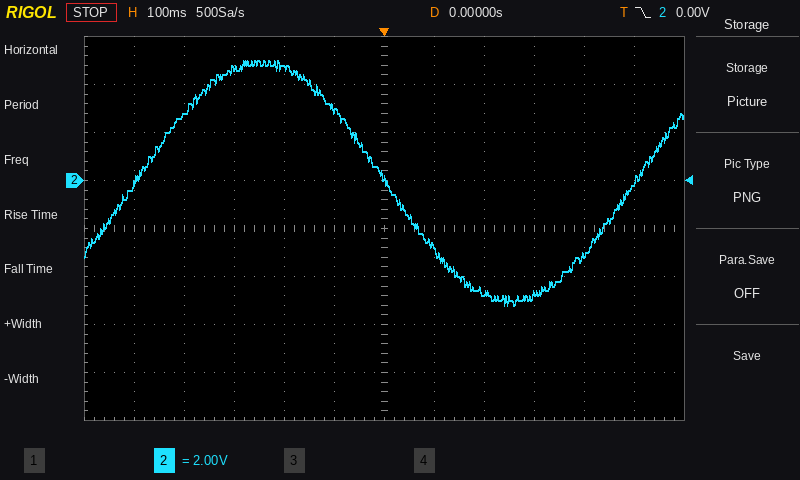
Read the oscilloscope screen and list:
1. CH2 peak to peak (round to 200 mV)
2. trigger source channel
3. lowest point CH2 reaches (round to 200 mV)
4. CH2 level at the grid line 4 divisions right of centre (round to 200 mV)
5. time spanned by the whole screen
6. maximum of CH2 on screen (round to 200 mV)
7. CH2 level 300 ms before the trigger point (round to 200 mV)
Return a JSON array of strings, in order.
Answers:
["10.2 V", "CH2", "-5.2 V", "-3.2 V", "1.2 s", "5.0 V", "4.6 V"]
